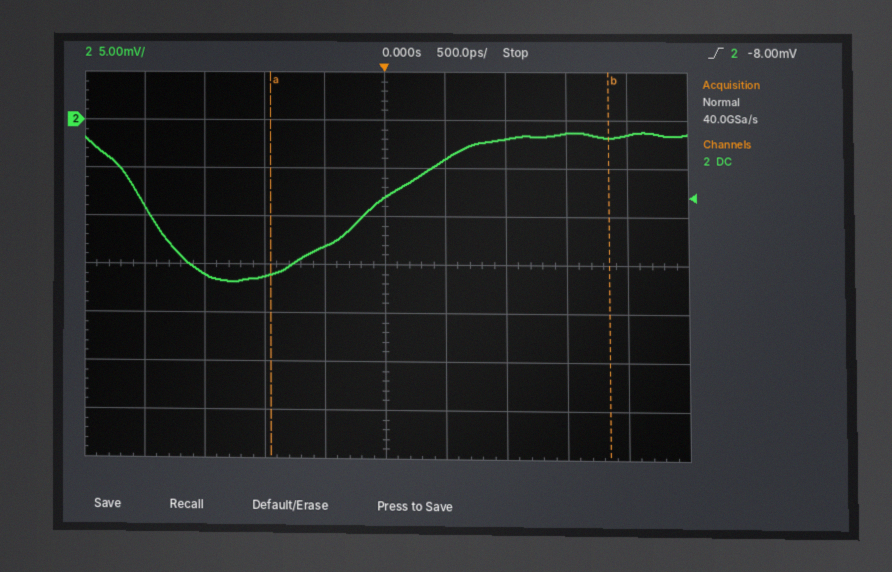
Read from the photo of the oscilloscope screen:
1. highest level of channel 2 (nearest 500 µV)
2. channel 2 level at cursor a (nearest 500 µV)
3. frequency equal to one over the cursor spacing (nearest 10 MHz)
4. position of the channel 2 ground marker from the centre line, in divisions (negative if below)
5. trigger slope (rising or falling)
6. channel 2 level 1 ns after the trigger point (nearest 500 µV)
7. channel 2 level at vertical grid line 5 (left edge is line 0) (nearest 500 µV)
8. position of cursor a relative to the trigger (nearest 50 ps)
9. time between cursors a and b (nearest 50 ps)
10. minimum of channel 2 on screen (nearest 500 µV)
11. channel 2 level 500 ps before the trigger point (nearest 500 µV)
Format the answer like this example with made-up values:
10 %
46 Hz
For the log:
-1.0 mV
-16.0 mV
360 MHz
+3.0 div
rising
-2.0 mV
-8.0 mV
-950 ps
2.80 ns
-17.0 mV
-13.0 mV
